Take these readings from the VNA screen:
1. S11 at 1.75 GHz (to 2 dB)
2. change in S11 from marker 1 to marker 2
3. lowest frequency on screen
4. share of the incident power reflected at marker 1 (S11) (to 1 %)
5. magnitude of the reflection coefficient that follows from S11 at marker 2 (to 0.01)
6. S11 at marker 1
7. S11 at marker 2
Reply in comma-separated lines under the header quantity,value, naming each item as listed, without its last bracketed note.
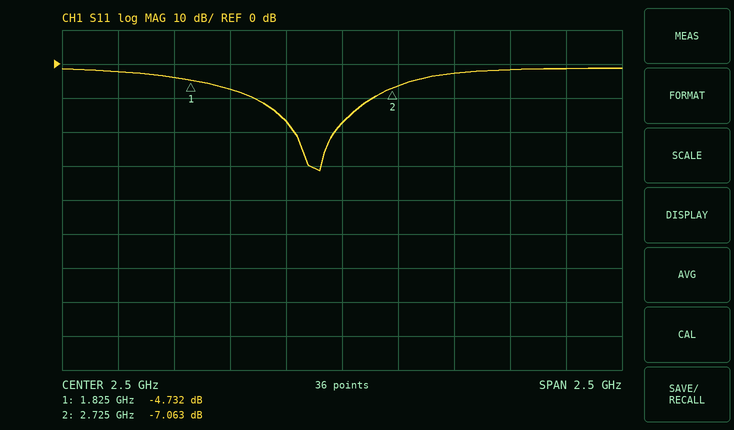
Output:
quantity,value
S11 at 1.75 GHz,-4 dB
change in S11 from marker 1 to marker 2,-2.331 dB
lowest frequency on screen,1.25 GHz
share of the incident power reflected at marker 1 (S11),34 %
magnitude of the reflection coefficient that follows from S11 at marker 2,0.44
S11 at marker 1,-4.732 dB
S11 at marker 2,-7.063 dB
